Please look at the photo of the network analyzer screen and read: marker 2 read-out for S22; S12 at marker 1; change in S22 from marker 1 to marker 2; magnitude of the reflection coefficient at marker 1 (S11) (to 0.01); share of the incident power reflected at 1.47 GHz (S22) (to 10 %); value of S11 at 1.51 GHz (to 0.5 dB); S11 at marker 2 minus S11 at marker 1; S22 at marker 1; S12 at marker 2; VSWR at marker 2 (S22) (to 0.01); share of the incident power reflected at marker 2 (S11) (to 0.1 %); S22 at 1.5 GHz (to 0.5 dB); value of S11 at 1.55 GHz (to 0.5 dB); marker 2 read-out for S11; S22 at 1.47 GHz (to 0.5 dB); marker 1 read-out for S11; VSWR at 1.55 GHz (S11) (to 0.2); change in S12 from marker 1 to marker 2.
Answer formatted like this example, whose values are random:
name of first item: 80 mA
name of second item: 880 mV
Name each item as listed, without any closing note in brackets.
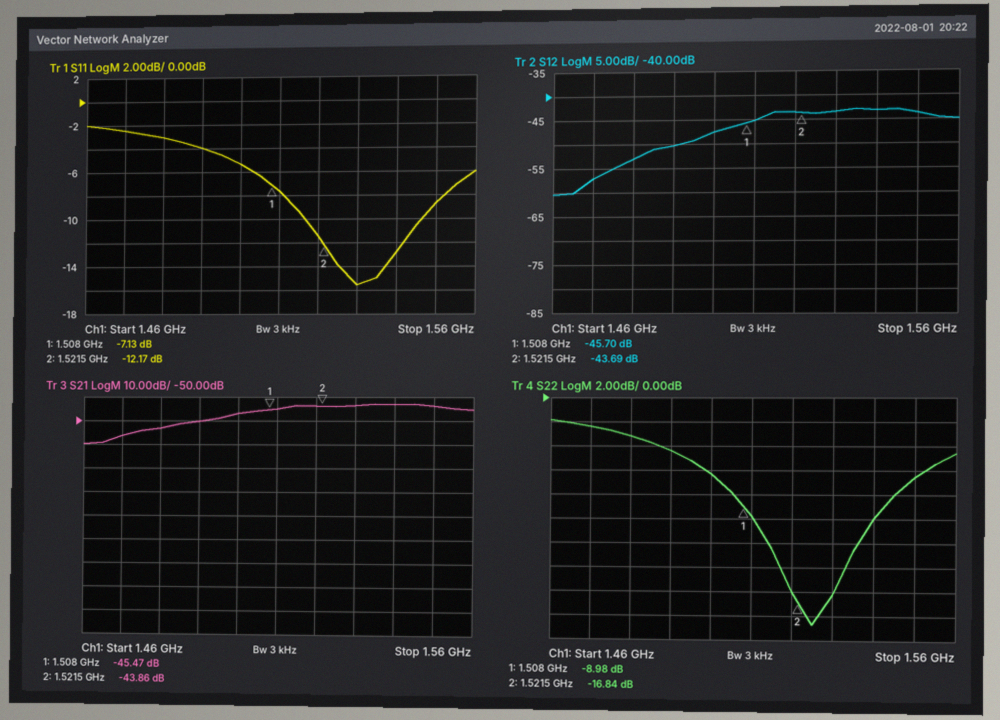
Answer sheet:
marker 2 read-out for S22: -16.84 dB
S12 at marker 1: -45.70 dB
change in S22 from marker 1 to marker 2: -7.86 dB
magnitude of the reflection coefficient at marker 1 (S11): 0.44
share of the incident power reflected at 1.47 GHz (S22): 60 %
value of S11 at 1.51 GHz: -7.5 dB
S11 at marker 2 minus S11 at marker 1: -5.04 dB
S22 at marker 1: -8.98 dB
S12 at marker 2: -43.69 dB
VSWR at marker 2 (S22): 1.34
share of the incident power reflected at marker 2 (S11): 6.1 %
S22 at 1.5 GHz: -6.5 dB
value of S11 at 1.55 GHz: -8.5 dB
marker 2 read-out for S11: -12.17 dB
S22 at 1.47 GHz: -2.5 dB
marker 1 read-out for S11: -7.13 dB
VSWR at 1.55 GHz (S11): 2.2
change in S12 from marker 1 to marker 2: 2.01 dB
